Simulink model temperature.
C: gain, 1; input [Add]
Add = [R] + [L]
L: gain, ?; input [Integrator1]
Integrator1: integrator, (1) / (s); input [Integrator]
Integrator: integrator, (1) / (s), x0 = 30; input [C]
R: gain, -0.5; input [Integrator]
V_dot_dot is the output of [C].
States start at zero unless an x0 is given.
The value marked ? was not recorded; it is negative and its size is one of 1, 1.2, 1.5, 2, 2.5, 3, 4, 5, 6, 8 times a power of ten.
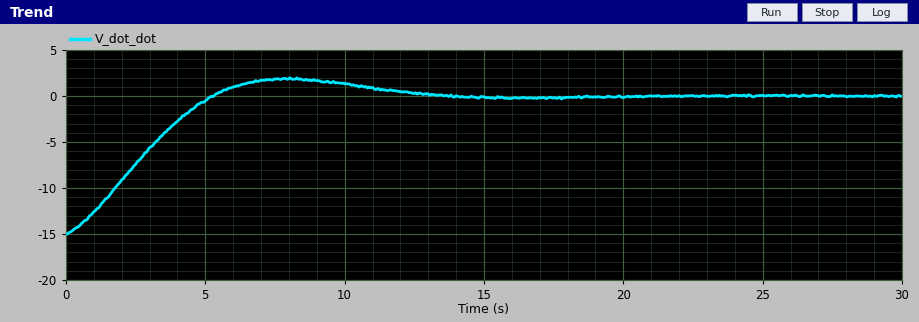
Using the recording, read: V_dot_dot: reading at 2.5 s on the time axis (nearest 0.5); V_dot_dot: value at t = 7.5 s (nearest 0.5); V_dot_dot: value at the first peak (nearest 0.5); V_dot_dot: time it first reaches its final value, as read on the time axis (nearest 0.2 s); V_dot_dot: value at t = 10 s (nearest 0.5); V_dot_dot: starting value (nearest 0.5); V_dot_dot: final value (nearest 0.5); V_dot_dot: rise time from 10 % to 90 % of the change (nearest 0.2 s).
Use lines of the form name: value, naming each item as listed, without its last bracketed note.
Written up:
V_dot_dot: reading at 2.5 s on the time axis: -7.5
V_dot_dot: value at t = 7.5 s: 2.0
V_dot_dot: value at the first peak: 2.0
V_dot_dot: time it first reaches its final value, as read on the time axis: 5.2 s
V_dot_dot: value at t = 10 s: 1.5
V_dot_dot: starting value: -15.0
V_dot_dot: final value: 0.0
V_dot_dot: rise time from 10 % to 90 % of the change: 3.8 s
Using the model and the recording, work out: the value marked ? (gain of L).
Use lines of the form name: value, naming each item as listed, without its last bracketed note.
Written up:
the value marked ?: -0.2
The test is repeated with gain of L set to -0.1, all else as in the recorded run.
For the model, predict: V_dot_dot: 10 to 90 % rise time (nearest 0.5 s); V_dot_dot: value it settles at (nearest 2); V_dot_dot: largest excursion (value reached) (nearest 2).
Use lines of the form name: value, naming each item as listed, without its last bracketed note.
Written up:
V_dot_dot: 10 to 90 % rise time: 4.5 s
V_dot_dot: value it settles at: 0
V_dot_dot: largest excursion (value reached): 0
